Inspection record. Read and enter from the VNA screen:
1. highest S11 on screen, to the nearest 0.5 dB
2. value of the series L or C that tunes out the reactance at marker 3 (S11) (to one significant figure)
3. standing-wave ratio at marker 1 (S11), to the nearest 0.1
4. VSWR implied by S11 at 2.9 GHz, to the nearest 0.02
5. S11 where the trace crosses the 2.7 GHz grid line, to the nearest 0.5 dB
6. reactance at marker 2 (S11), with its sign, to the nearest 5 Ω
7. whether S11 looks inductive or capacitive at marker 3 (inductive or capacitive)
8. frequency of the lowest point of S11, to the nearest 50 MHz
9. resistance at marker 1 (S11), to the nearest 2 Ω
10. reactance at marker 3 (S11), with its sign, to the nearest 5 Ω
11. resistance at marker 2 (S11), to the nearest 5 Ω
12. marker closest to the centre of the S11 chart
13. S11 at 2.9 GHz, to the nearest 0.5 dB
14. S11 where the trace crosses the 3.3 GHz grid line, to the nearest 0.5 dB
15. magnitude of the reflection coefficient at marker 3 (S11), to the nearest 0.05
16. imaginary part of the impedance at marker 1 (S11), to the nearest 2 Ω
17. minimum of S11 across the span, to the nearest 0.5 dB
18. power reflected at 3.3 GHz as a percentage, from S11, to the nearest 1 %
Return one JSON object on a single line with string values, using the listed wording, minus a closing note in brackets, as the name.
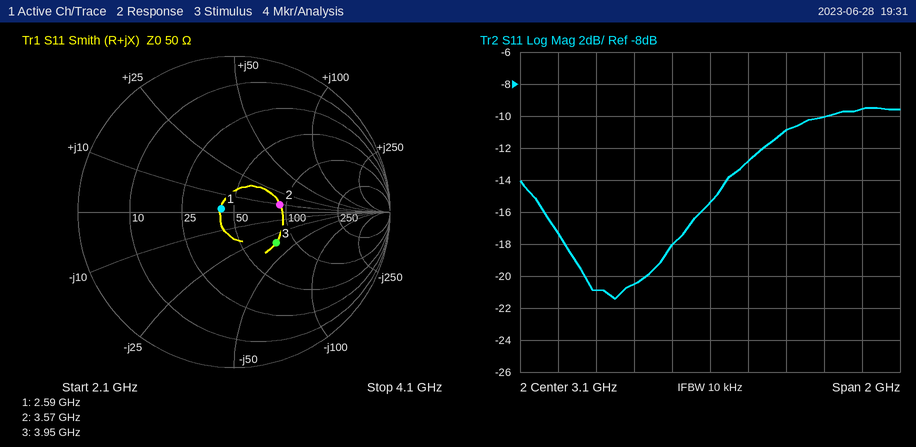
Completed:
{"highest S11 on screen, to the nearest 0.5 dB": "-9.5 dB", "value of the series L or C that tunes out the reactance at marker 3 (S11)": "1 nH", "standing-wave ratio at marker 1 (S11), to the nearest 0.1": "1.2", "VSWR implied by S11 at 2.9 GHz, to the nearest 0.02": "1.28", "S11 where the trace crosses the 2.7 GHz grid line, to the nearest 0.5 dB": "-20.5 dB", "reactance at marker 2 (S11), with its sign, to the nearest 5 Ω": "+10 Ω", "whether S11 looks inductive or capacitive at marker 3": "capacitive", "frequency of the lowest point of S11, to the nearest 50 MHz": "2.60 GHz", "resistance at marker 1 (S11), to the nearest 2 Ω": "42 Ω", "reactance at marker 3 (S11), with its sign, to the nearest 5 Ω": "-35 Ω", "resistance at marker 2 (S11), to the nearest 5 Ω": "90 Ω", "marker closest to the centre of the S11 chart": "marker 1", "S11 at 2.9 GHz, to the nearest 0.5 dB": "-18.0 dB", "S11 where the trace crosses the 3.3 GHz grid line, to the nearest 0.5 dB": "-13.0 dB", "magnitude of the reflection coefficient at marker 3 (S11), to the nearest 0.05": "0.35", "imaginary part of the impedance at marker 1 (S11), to the nearest 2 Ω": "+2 Ω", "minimum of S11 across the span, to the nearest 0.5 dB": "-21.5 dB", "power reflected at 3.3 GHz as a percentage, from S11, to the nearest 1 %": "5 %"}
